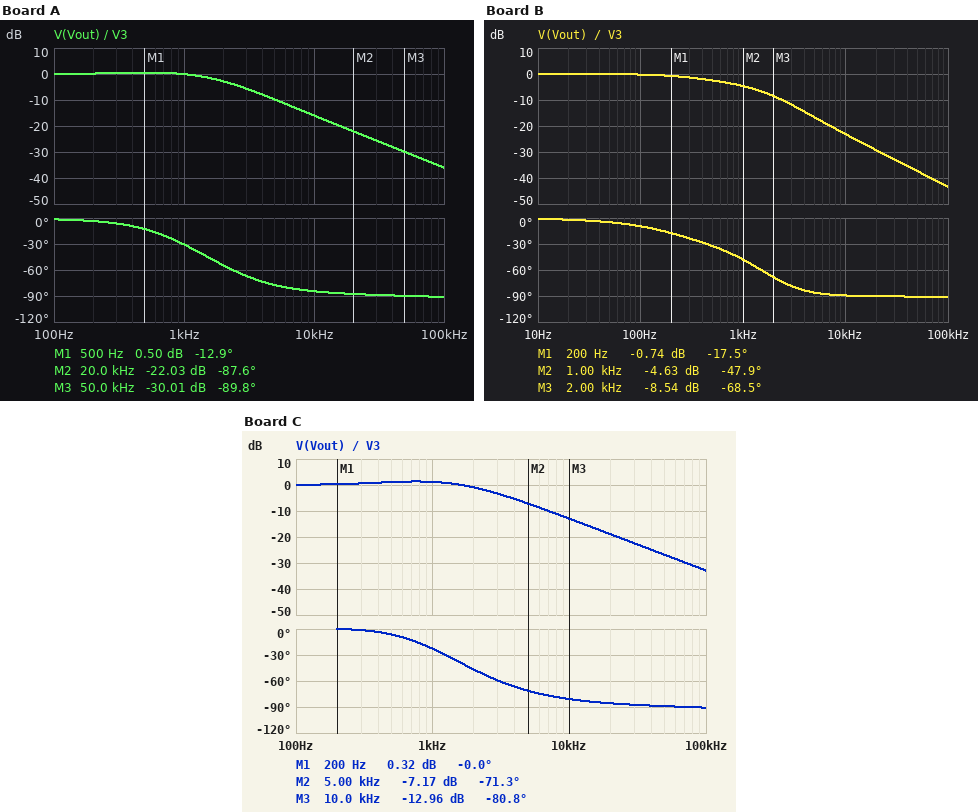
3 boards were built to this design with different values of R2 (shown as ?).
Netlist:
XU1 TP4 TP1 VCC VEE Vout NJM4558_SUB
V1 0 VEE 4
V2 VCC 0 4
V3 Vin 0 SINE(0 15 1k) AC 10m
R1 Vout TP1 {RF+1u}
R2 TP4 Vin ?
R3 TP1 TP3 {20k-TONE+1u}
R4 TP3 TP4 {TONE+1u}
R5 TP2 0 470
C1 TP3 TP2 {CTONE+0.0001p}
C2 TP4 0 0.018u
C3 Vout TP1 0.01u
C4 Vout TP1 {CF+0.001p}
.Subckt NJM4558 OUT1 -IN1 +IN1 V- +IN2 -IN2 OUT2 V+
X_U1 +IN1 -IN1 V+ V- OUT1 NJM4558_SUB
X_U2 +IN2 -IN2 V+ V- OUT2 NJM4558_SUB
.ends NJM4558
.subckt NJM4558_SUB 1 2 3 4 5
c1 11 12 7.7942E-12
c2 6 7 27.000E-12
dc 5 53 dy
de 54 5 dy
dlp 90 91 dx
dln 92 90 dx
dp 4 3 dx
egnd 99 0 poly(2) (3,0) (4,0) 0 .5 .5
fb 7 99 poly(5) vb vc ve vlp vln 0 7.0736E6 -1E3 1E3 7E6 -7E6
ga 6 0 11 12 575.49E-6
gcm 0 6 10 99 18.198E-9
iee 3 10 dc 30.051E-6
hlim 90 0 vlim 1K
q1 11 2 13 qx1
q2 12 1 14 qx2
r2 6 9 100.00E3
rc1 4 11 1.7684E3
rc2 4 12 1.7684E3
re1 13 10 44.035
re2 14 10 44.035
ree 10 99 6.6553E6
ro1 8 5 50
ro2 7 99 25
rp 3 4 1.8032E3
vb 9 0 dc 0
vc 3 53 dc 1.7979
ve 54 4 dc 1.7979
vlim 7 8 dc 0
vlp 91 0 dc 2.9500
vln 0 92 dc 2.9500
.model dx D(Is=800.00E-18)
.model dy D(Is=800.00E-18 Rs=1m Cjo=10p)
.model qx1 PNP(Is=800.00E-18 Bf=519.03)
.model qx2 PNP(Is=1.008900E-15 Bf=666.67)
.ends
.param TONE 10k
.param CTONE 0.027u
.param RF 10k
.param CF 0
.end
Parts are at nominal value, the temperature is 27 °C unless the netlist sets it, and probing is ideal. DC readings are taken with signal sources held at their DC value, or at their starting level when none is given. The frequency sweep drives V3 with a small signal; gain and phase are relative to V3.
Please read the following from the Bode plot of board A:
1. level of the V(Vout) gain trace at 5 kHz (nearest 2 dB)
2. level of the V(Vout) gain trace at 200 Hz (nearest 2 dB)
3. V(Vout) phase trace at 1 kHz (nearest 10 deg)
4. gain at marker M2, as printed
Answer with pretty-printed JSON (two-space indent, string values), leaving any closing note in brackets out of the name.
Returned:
{
  "level of the V(Vout) gain trace at 5 kHz": "-10 dB",
  "level of the V(Vout) gain trace at 200 Hz": "0 dB",
  "V(Vout) phase trace at 1 kHz": "-30 deg",
  "gain at marker M2, as printed": "-22.03 dB"
}
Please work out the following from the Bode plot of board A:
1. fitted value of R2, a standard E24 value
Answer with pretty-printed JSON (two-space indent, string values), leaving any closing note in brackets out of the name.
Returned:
{
  "fitted value of R2, a standard E24 value": "5.6 kΩ"
}
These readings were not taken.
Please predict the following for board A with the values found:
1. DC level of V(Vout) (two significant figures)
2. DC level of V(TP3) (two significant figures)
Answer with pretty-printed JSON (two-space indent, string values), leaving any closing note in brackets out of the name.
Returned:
{
  "DC level of V(Vout)": "-11 mV",
  "DC level of V(TP3)": "-4.6 mV"
}
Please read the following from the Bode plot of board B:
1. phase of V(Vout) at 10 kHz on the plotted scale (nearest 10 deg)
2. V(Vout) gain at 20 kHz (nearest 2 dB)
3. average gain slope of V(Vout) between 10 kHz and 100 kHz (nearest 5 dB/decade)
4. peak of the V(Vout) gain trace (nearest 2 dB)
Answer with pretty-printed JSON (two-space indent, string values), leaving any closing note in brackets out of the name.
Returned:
{
  "phase of V(Vout) at 10 kHz on the plotted scale": "-90 deg",
  "V(Vout) gain at 20 kHz": "-30 dB",
  "average gain slope of V(Vout) between 10 kHz and 100 kHz": "-20 dB/decade",
  "peak of the V(Vout) gain trace": "0 dB"
}
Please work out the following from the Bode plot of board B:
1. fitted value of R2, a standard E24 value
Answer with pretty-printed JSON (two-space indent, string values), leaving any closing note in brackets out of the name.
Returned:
{
  "fitted value of R2, a standard E24 value": "13 kΩ"
}
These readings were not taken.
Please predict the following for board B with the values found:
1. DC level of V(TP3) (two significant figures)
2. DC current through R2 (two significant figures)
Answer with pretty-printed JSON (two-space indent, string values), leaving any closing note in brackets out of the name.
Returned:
{
  "DC level of V(TP3)": "-6.6 mV",
  "DC current through R2": "280 nA"
}
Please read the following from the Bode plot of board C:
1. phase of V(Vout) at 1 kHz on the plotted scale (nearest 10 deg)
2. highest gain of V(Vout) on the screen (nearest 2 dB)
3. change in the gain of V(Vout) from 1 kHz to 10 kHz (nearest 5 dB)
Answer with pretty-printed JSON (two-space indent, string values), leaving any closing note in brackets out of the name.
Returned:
{
  "phase of V(Vout) at 1 kHz on the plotted scale": "-20 deg",
  "highest gain of V(Vout) on the screen": "2 dB",
  "change in the gain of V(Vout) from 1 kHz to 10 kHz": "-15 dB"
}
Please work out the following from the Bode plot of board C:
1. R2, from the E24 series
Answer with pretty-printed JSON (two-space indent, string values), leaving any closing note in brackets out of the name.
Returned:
{
  "R2, from the E24 series": "3.9 kΩ"
}
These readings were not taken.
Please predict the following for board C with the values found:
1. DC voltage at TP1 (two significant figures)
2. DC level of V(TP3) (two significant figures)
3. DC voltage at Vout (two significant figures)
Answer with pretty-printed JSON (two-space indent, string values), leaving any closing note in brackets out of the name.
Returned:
{
  "DC voltage at TP1": "-7.1 mV",
  "DC level of V(TP3)": "-4.1 mV",
  "DC voltage at Vout": "-10 mV"
}
